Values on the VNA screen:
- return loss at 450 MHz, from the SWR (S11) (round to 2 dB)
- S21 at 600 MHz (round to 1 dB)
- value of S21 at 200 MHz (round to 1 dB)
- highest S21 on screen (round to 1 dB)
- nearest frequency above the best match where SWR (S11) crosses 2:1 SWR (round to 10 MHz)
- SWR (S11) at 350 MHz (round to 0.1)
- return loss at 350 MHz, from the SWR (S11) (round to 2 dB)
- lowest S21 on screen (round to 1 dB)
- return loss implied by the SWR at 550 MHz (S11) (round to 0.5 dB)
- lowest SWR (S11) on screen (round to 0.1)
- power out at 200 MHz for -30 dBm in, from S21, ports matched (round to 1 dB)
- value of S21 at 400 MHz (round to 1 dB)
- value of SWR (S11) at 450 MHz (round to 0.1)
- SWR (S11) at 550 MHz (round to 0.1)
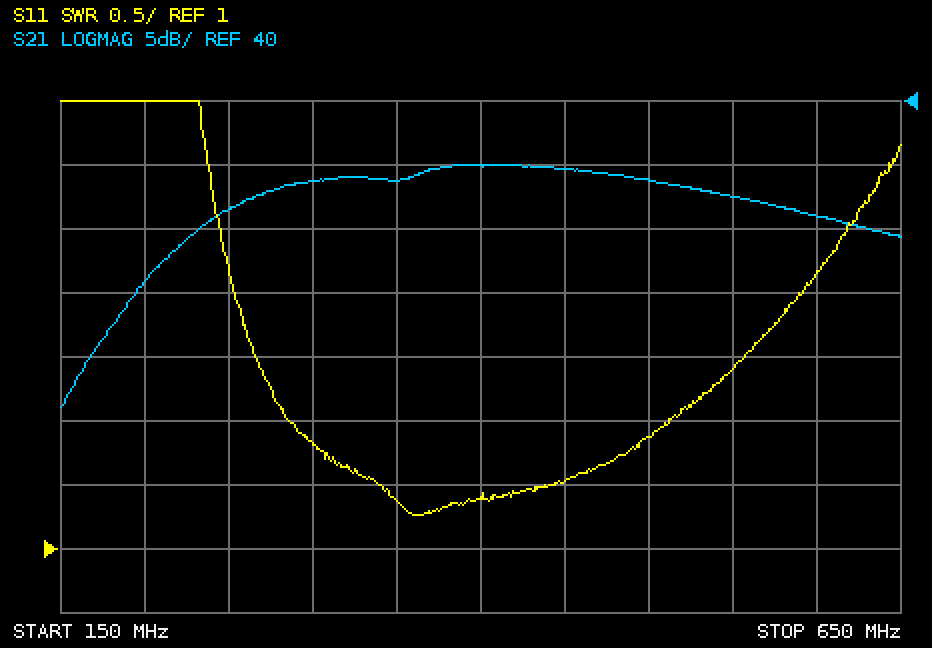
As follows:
14 dB
31 dB
26 dB
35 dB
510 MHz
1.4
16 dB
16 dB
7.5 dB
1.3
-4 dBm
35 dB
1.5
2.4
